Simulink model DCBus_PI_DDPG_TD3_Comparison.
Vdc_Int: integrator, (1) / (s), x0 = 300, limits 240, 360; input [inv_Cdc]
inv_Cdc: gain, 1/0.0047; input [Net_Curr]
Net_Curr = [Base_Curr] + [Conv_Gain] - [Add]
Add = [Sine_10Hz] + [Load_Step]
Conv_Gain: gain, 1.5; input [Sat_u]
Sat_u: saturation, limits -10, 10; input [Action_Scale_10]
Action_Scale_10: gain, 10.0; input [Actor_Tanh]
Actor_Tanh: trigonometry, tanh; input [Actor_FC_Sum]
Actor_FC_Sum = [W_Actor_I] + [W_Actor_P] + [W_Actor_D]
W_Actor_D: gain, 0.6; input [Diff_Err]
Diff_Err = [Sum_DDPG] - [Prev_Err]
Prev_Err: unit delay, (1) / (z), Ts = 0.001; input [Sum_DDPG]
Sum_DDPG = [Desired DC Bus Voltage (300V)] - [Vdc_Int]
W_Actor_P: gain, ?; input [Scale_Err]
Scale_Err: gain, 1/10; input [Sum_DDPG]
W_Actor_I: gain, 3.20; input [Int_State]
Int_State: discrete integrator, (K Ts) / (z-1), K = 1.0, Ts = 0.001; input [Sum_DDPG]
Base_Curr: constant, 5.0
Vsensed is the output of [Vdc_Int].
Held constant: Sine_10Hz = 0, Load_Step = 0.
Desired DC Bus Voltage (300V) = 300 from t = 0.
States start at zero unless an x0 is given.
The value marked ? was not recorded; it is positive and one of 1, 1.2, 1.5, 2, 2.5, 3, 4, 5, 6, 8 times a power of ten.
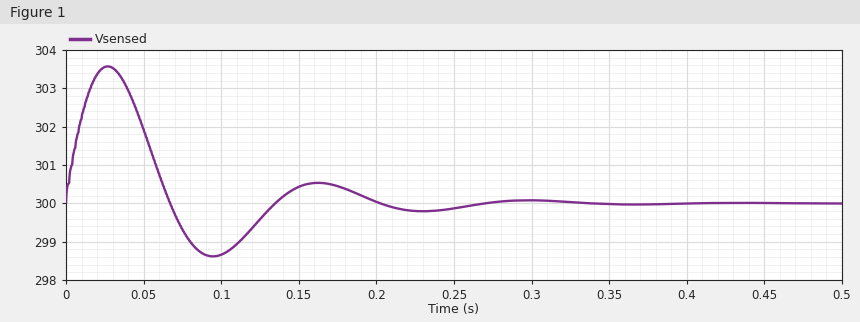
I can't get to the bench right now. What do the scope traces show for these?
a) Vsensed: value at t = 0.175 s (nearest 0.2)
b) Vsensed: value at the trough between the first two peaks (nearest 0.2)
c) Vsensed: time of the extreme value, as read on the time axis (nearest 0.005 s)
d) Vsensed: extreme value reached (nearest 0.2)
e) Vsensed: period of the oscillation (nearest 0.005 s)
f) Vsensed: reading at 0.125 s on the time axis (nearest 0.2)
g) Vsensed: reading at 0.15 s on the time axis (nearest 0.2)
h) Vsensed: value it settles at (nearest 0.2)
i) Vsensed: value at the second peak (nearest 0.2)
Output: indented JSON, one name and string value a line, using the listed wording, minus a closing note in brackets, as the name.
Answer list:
{
  "Vsensed: value at t = 0.175 s": "300.4",
  "Vsensed: value at the trough between the first two peaks": "298.6",
  "Vsensed: time of the extreme value, as read on the time axis": "0.025 s",
  "Vsensed: extreme value reached": "303.6",
  "Vsensed: period of the oscillation": "0.135 s",
  "Vsensed: reading at 0.125 s on the time axis": "299.6",
  "Vsensed: reading at 0.15 s on the time axis": "300.4",
  "Vsensed: value it settles at": "300.0",
  "Vsensed: value at the second peak": "300.6"
}
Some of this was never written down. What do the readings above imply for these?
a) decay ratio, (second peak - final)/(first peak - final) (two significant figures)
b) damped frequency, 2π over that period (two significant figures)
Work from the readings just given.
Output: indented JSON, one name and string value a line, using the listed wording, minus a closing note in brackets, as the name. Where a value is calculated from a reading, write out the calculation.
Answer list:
{
  "decay ratio, (second peak - final)/(first peak - final)": "(300.6 - 300) / (303.6 - 300) = 0.17",
  "damped frequency, 2π over that period": "2π / 0.135 = 47 rad/s"
}
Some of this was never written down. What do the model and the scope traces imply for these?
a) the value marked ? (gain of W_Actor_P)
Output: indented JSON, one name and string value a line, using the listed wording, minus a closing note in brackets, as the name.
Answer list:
{
  "the value marked ?": "0.4"
}
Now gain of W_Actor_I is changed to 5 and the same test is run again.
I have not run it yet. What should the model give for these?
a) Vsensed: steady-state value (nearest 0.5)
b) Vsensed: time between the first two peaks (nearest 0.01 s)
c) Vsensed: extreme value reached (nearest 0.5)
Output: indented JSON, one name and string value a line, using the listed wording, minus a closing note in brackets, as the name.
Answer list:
{
  "Vsensed: steady-state value": "300.0",
  "Vsensed: time between the first two peaks": "0.11 s",
  "Vsensed: extreme value reached": "303.0"
}
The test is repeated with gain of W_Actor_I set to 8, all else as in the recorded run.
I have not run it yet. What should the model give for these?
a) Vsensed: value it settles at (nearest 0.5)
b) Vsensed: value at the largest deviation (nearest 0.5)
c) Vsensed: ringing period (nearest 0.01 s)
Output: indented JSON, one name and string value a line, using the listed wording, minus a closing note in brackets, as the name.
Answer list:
{
  "Vsensed: value it settles at": "300.0",
  "Vsensed: value at the largest deviation": "302.5",
  "Vsensed: ringing period": "0.08 s"
}
